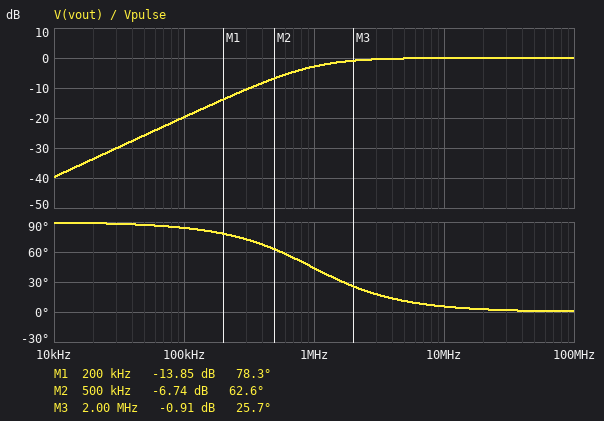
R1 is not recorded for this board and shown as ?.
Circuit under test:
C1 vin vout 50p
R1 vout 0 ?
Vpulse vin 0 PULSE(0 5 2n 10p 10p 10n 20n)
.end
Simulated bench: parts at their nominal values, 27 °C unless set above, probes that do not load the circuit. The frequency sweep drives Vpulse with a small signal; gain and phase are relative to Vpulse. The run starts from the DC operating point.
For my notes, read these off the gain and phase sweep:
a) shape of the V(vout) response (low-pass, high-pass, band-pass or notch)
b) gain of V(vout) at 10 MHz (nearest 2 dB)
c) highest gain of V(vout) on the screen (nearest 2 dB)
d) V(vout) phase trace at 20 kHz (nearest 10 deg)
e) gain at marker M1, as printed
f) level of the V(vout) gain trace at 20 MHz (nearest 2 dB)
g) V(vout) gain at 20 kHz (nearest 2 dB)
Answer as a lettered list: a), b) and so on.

a) high-pass
b) 0 dB
c) 0 dB
d) 90 deg
e) -13.85 dB
f) 0 dB
g) -34 dB
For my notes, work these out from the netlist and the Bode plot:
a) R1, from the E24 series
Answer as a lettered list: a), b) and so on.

a) 3.3 kΩ
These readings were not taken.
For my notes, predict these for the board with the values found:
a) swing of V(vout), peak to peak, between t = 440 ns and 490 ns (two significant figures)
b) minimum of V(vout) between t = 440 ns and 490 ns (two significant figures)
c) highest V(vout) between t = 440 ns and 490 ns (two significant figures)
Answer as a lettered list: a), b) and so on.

a) 5.2 V
b) -2.4 V
c) 2.7 V
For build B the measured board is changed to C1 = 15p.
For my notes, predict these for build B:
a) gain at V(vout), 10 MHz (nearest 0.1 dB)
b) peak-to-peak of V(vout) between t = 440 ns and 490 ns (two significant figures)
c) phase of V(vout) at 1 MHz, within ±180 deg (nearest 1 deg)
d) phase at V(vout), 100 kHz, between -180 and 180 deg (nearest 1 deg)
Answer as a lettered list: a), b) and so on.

a) -0.4 dB
b) 5.5 V
c) 73 deg
d) 88 deg
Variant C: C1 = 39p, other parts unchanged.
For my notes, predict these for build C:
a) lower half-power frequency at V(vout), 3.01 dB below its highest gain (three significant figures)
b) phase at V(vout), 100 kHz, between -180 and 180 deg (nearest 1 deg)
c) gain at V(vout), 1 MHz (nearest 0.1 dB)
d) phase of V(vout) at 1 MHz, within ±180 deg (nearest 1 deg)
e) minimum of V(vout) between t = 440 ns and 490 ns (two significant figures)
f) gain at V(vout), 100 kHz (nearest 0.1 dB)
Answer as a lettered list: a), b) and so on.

a) 1.24 MHz
b) 85 deg
c) -4.0 dB
d) 51 deg
e) -2.5 V
f) -21.9 dB
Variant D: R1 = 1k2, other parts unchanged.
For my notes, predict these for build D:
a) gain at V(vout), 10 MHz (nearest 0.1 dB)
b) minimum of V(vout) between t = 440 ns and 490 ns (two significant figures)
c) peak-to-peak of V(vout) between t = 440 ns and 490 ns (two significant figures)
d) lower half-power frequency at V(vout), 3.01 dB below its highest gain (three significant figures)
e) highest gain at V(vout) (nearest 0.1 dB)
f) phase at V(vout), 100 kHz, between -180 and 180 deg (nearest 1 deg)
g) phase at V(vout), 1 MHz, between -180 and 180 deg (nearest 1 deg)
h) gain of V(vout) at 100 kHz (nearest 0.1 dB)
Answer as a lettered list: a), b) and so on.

a) -0.3 dB
b) -2.7 V
c) 5.4 V
d) 2.65 MHz
e) 0 dB
f) 88 deg
g) 69 deg
h) -28.5 dB
